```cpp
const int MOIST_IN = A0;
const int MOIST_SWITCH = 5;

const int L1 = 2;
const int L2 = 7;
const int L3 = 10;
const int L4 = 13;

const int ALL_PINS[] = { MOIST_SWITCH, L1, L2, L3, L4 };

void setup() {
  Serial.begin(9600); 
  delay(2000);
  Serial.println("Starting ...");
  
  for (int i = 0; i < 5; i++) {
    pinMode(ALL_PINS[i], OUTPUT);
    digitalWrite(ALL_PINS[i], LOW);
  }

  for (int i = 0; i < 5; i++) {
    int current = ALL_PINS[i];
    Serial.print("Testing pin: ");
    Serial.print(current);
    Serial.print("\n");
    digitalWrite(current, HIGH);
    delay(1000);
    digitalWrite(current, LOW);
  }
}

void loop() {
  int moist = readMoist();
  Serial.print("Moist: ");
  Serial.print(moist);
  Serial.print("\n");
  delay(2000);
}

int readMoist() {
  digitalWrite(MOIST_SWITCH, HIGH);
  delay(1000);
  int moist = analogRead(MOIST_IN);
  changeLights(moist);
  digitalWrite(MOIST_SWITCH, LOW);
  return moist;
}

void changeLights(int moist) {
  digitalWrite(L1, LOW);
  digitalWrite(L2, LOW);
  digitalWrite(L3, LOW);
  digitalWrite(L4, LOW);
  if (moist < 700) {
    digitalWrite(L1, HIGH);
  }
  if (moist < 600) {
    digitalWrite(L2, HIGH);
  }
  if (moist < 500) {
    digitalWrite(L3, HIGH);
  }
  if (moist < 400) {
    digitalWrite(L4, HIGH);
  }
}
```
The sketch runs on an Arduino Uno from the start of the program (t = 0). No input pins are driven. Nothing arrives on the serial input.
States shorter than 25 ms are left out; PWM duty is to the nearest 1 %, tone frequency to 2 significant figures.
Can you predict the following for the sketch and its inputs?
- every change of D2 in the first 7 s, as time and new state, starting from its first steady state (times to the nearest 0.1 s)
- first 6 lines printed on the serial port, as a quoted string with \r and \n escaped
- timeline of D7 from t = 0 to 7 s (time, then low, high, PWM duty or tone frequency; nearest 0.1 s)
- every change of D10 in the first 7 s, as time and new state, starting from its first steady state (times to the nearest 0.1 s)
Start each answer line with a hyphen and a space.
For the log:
- 2 s low; 3 s high; 4 s low
- "Starting ...\r\nTesting pin: 5\nTesting pin: 2\nTesting pin: 7\nTesting pin: 10\nTesting pin: 13\n"
- 2 s low; 4 s high; 5 s low
- 2 s low; 5 s high; 6 s low
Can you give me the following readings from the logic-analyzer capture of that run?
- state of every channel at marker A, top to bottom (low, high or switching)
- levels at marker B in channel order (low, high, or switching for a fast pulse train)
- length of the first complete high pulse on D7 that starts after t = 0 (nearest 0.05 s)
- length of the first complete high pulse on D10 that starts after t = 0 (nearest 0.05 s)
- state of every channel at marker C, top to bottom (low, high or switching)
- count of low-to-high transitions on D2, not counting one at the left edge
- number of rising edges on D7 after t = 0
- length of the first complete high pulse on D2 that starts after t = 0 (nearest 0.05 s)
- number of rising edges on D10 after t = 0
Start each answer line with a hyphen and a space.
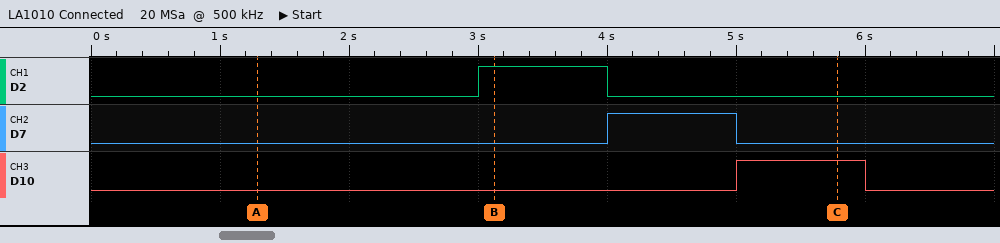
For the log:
- D2 low, D7 low, D10 low
- D2 high, D7 low, D10 low
- 1.00 s
- 1.00 s
- D2 low, D7 low, D10 high
- 1
- 1
- 1.00 s
- 1
